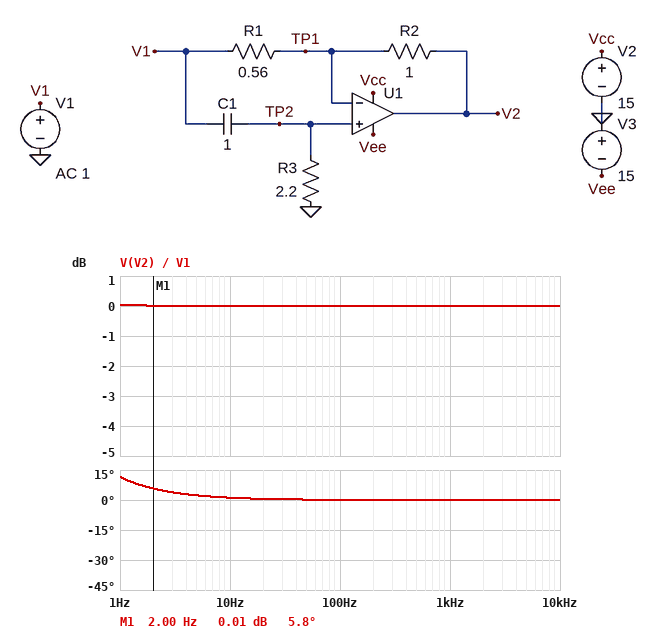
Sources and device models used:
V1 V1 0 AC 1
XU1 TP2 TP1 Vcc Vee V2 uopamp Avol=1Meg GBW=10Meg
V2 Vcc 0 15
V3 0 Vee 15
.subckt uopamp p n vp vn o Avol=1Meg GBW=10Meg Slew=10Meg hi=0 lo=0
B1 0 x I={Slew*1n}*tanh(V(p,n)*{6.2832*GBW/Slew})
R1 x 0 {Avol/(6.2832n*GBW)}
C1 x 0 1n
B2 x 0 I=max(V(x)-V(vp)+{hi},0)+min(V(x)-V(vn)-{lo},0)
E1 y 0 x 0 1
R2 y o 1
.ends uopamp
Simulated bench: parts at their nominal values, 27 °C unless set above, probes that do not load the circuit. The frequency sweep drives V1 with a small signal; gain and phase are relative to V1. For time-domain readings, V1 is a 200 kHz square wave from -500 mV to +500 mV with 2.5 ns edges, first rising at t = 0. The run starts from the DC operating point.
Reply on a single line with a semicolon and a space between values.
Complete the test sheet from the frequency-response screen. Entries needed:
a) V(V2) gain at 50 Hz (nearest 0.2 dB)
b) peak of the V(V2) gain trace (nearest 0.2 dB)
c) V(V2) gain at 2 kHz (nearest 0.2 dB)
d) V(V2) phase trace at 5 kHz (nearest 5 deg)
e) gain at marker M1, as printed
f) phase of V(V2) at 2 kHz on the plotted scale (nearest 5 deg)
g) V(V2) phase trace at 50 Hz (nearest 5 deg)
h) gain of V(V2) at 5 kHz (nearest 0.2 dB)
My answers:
0 dB; 0 dB; 0 dB; 0 deg; 0.01 dB; 0 deg; 0 deg; 0 dB
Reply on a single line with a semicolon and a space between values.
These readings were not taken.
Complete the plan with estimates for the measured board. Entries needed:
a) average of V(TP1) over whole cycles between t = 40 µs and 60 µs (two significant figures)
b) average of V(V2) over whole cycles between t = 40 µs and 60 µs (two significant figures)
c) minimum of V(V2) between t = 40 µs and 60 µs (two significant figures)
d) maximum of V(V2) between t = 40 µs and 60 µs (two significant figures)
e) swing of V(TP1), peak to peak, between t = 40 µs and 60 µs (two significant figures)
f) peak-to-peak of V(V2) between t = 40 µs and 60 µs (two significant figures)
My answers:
500 mV; 1.4 V; 890 mV; 1.9 V; 1.0 V; 1.0 V
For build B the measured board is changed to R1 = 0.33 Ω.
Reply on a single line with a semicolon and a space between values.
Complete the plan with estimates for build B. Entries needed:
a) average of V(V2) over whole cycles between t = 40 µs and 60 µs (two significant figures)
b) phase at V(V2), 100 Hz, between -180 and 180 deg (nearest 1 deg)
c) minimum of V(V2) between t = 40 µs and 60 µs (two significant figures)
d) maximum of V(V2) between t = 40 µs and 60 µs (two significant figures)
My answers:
2.0 V; 0 deg; 1.5 V; 2.5 V
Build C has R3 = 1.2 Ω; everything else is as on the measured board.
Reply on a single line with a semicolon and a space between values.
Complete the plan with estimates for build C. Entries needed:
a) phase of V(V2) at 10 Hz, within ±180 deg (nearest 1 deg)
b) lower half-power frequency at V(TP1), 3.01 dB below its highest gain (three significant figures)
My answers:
2 deg; 133 mHz
